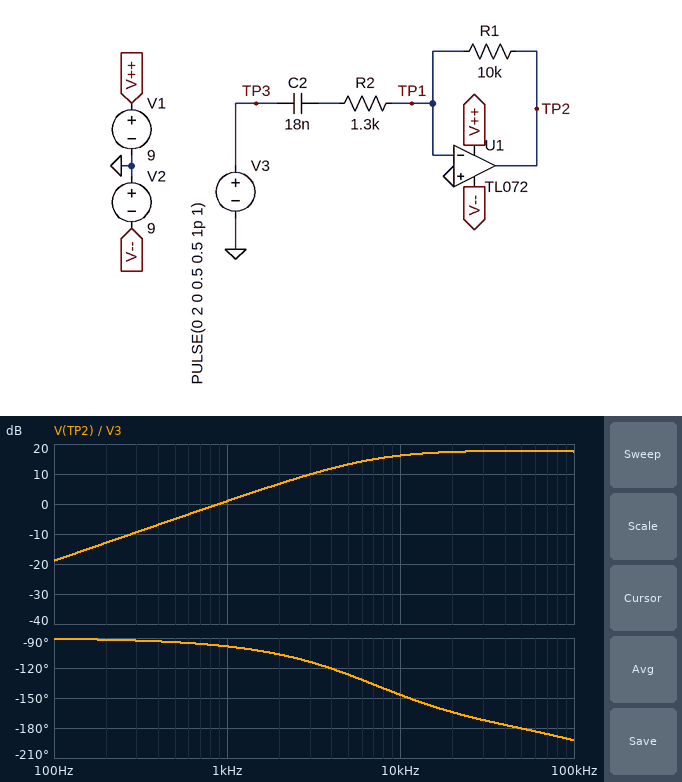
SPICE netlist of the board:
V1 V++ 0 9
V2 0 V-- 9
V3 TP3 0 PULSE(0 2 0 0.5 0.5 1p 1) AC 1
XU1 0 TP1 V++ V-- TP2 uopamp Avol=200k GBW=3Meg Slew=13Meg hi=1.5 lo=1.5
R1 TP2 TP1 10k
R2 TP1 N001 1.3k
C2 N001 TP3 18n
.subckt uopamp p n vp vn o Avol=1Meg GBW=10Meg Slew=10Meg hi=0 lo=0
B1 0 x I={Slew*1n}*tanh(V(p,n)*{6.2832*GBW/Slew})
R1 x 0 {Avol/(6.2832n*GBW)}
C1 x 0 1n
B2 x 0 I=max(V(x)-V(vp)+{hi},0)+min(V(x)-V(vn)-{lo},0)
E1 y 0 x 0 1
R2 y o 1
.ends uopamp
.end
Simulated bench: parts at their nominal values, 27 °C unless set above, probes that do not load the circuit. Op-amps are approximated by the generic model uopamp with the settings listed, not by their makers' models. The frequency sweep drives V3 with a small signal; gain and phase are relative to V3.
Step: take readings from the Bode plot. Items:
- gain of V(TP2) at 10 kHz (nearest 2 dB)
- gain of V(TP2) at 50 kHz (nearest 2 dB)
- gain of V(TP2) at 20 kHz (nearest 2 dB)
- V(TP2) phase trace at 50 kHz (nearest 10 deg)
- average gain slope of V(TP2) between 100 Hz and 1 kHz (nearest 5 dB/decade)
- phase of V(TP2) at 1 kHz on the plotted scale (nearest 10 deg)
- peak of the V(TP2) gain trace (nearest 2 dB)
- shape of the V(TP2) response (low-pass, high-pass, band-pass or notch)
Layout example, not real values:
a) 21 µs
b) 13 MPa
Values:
a) 16 dB
b) 18 dB
c) 18 dB
d) -180 deg
e) 20 dB/decade
f) -100 deg
g) 18 dB
h) high-pass
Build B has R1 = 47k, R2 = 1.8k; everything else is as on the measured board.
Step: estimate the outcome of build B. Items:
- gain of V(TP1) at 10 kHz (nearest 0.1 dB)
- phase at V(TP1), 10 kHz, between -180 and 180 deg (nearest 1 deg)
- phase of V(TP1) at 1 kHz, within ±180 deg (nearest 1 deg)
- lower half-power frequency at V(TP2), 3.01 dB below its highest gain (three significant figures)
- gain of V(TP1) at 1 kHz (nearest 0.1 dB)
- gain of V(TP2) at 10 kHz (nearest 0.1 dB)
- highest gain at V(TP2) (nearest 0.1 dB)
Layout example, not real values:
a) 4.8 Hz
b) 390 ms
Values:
a) -21.9 dB
b) 112 deg
c) 168 deg
d) 4.70 kHz
e) -55.2 dB
f) 27.7 dB
g) 28.3 dB
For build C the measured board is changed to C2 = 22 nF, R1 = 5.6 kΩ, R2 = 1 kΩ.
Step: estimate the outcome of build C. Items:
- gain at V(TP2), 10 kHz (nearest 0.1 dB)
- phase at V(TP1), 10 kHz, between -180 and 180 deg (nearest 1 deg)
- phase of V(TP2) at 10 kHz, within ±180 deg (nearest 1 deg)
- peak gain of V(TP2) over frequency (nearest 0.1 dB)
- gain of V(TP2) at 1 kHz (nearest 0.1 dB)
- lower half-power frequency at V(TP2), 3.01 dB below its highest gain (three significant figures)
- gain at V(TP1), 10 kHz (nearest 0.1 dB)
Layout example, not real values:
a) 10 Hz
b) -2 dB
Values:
a) 13.2 dB
b) 125 deg
c) -145 deg
d) 14.9 dB
e) -2.3 dB
f) 7.11 kHz
g) -36.3 dB
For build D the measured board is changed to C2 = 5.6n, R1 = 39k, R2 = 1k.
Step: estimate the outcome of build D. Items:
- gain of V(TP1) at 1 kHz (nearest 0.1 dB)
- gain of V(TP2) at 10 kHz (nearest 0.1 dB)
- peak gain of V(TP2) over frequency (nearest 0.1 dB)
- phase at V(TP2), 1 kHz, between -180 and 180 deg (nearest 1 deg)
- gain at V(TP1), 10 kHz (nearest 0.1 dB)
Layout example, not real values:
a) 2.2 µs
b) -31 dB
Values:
a) -66.8 dB
b) 22.6 dB
c) 31.7 dB
d) -92 deg
e) -26.9 dB
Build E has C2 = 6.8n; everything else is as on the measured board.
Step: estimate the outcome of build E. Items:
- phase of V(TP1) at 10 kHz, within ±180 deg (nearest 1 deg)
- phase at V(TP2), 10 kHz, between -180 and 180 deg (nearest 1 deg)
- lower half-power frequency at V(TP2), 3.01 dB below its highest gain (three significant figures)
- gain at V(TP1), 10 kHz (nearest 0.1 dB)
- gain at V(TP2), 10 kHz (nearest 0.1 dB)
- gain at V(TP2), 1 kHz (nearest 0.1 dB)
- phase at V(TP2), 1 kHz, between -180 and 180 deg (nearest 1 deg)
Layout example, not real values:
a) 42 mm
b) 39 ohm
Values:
a) 150 deg
b) -120 deg
c) 17.1 kHz
d) -38.0 dB
e) 11.5 dB
f) -7.4 dB
g) -93 deg
